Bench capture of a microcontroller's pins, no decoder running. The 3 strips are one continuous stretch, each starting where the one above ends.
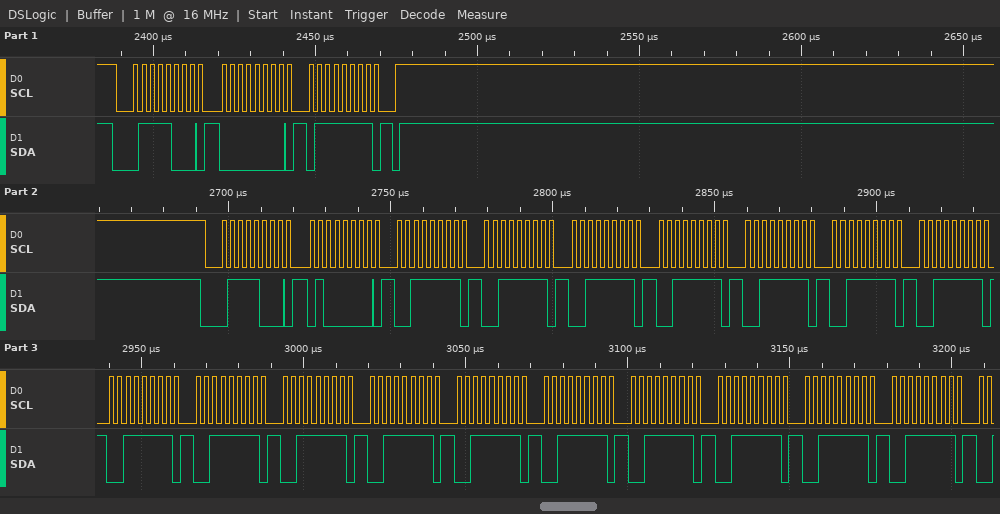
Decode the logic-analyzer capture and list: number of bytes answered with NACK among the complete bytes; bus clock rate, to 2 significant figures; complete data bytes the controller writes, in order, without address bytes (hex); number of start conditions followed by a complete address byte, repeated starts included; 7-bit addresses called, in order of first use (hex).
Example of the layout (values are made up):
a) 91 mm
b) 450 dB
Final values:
a) 0
b) 400 kHz
c) 00 7F 40 3F 3F 3F 3F 3F 3F 3F 3F 3F 3F 3F 3F 3F 3F 3F 3F 3F
d) 2
e) 0x3C
